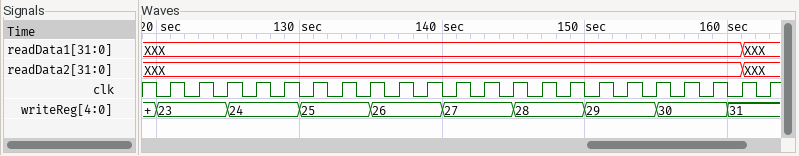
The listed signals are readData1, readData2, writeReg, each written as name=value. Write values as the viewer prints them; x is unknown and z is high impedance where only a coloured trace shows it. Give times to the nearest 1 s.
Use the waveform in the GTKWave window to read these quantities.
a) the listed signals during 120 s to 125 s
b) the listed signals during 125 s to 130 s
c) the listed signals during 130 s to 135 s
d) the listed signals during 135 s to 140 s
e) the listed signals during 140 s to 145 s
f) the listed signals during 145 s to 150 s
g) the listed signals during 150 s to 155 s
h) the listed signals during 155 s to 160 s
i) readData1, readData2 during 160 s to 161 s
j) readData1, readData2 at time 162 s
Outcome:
readData1=XXX, readData2=XXX, writeReg=23
readData1=XXX, readData2=XXX, writeReg=24
readData1=XXX, readData2=XXX, writeReg=25
readData1=XXX, readData2=XXX, writeReg=26
readData1=XXX, readData2=XXX, writeReg=27
readData1=XXX, readData2=XXX, writeReg=28
readData1=XXX, readData2=XXX, writeReg=29
readData1=XXX, readData2=XXX, writeReg=30
readData1=XXX, readData2=XXX
readData1=XXX, readData2=XXX
